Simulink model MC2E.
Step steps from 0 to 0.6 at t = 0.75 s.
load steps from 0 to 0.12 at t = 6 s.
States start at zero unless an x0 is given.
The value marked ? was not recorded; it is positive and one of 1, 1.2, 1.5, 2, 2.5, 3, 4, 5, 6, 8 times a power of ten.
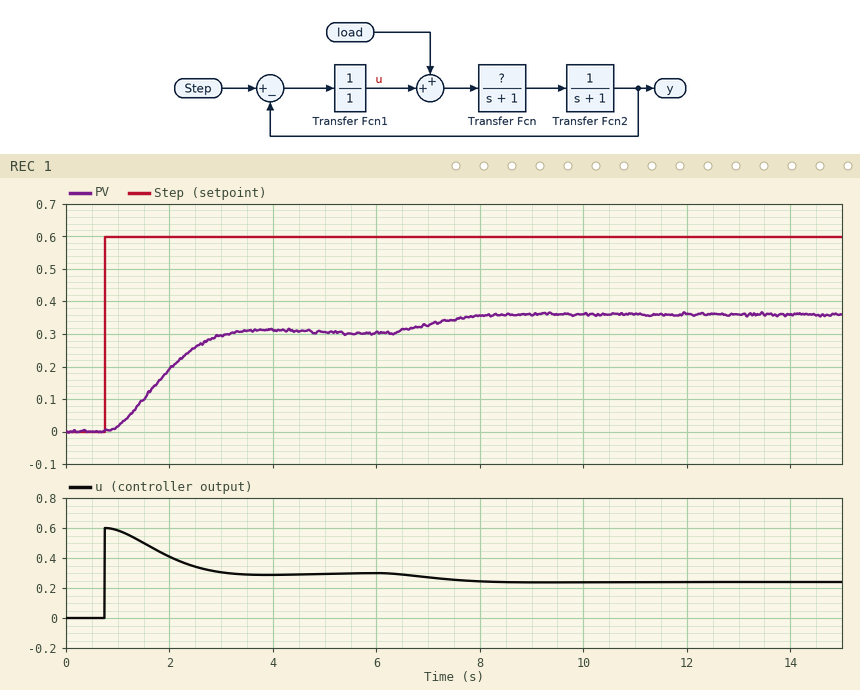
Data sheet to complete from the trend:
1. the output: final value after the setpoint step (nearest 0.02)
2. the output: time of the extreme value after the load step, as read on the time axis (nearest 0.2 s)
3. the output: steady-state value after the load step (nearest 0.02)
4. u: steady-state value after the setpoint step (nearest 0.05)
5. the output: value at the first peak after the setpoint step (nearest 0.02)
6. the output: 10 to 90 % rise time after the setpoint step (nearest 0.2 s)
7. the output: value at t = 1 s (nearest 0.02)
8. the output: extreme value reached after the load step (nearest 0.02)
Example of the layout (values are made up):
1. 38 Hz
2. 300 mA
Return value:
1. 0.30
2. 9.2 s
3. 0.36
4. 0.30
5. 0.32
6. 1.6 s
7. 0.02
8. 0.36
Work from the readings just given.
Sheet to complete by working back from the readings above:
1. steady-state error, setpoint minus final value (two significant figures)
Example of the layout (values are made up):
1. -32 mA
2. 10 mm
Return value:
1. 0.30
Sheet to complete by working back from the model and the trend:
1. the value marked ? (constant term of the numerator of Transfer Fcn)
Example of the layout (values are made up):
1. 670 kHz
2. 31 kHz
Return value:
1. 1
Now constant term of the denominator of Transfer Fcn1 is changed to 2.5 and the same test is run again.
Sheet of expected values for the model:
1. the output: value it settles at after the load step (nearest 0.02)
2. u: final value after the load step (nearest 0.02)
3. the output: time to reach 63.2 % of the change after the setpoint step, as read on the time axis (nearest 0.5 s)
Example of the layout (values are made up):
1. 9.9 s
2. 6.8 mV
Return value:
1. 0.26
2. 0.14
3. 2.5 s
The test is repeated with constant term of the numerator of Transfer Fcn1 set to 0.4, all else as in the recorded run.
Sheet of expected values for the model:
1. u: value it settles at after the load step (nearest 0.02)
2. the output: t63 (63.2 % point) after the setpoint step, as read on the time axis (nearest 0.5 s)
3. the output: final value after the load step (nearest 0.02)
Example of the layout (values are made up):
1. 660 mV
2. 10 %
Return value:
1. 0.14
2. 2.5 s
3. 0.26
